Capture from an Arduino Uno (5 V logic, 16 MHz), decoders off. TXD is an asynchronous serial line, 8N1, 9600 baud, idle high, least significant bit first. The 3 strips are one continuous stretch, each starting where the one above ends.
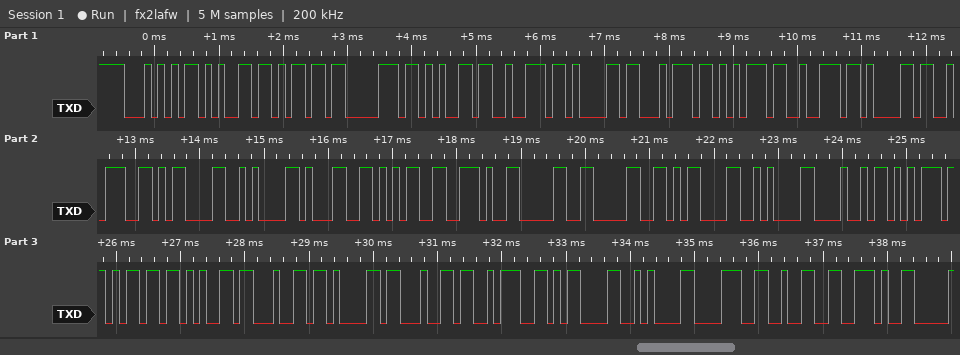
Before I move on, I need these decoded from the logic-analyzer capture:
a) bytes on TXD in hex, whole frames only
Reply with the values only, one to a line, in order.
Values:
54 65 6D 70 65 72 61 74 75 72 61 3A 0D 0A 31 35 2E 30 30 0D 0A 48 75 6D 65 64 61 64 3A 0D 0A 38 32 2E
